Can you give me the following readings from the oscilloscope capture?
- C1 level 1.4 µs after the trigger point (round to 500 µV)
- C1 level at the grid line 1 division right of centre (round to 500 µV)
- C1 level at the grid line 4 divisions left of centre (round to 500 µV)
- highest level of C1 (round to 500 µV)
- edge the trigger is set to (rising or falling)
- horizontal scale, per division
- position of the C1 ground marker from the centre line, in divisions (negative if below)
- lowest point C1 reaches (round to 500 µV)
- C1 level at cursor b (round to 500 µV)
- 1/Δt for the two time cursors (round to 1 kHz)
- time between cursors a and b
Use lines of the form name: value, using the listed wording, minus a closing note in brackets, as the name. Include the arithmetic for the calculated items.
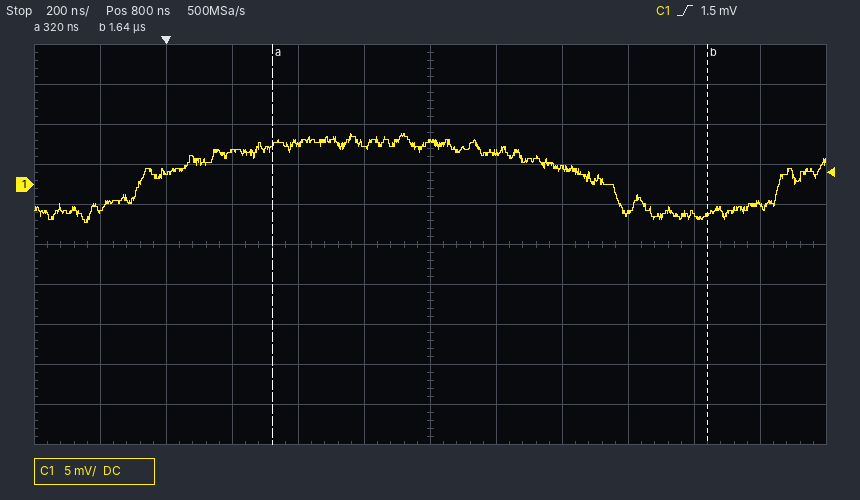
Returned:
C1 level 1.4 µs after the trigger point: -3.5 mV
C1 level at the grid line 1 division right of centre: 4.0 mV
C1 level at the grid line 4 divisions left of centre: 1.5 mV
highest level of C1: 6.5 mV
edge the trigger is set to: rising
horizontal scale, per division: 200 ns
position of the C1 ground marker from the centre line, in divisions: +1.5 div
lowest point C1 reaches: -5.0 mV
C1 level at cursor b: -3.5 mV
1/Δt for the two time cursors: 1 / 1.32 µs ≈ 758 kHz
time between cursors a and b: 1.64 µs − (320 ns) = 1.32 µs
